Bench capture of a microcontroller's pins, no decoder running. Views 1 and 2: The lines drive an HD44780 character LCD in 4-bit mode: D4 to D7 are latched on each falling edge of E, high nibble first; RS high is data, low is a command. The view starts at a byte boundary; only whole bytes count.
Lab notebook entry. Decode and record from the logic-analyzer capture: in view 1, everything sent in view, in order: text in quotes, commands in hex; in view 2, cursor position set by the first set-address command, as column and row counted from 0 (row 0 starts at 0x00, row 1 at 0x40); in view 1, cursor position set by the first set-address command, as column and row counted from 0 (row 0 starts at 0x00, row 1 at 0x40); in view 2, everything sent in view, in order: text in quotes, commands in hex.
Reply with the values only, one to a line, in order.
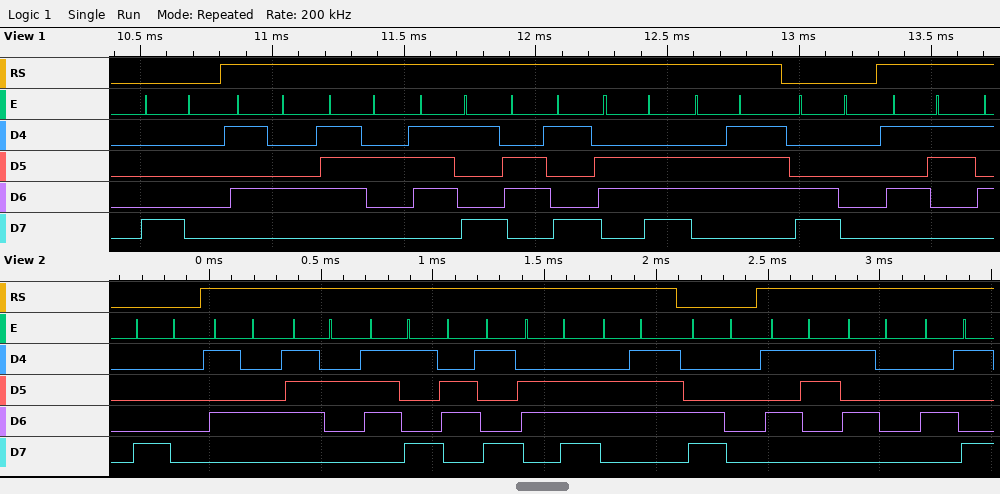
0x80 "Trying" 0xC0 "S"
column 0, row 0
column 0, row 0
0x80 "Trying" 0xC0 "SPI"
